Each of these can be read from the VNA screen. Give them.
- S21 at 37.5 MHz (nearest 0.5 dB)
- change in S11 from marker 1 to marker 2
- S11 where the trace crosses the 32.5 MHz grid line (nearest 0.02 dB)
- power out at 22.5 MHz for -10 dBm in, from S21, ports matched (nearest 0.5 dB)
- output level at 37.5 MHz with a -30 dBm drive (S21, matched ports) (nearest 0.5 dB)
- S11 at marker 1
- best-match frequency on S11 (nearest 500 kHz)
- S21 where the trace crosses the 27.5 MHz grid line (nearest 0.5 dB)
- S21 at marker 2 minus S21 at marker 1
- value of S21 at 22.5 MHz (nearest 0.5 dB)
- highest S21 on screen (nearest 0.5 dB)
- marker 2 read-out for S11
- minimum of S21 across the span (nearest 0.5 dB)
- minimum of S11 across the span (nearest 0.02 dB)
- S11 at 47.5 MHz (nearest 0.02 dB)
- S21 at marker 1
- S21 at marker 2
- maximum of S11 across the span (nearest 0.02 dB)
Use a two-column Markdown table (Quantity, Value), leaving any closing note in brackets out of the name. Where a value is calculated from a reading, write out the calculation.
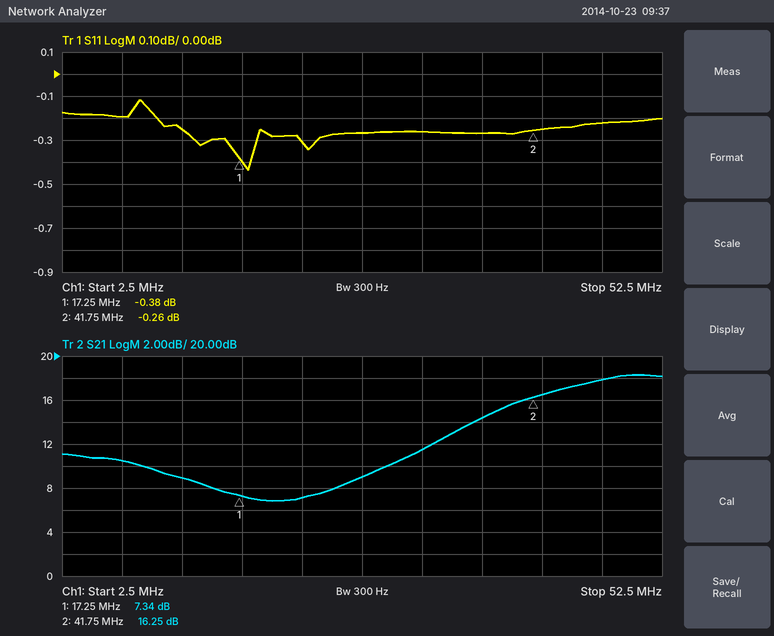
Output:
| Quantity | Value |
|---|---|
| S21 at 37.5 MHz | 14.5 dB |
| change in S11 from marker 1 to marker 2 | -0.26 − (-0.38) = 0.12 dB |
| S11 where the trace crosses the 32.5 MHz grid line | -0.26 dB |
| power out at 22.5 MHz for -10 dBm in, from S21, ports matched | -10 dBm + (7.0 dB) = -3.0 dBm |
| output level at 37.5 MHz with a -30 dBm drive (S21, matched ports) | -30 dBm + (14.5 dB) = -15.5 dBm |
| S11 at marker 1 | -0.38 dB |
| best-match frequency on S11 | 18.0 MHz |
| S21 where the trace crosses the 27.5 MHz grid line | 9.0 dB |
| S21 at marker 2 minus S21 at marker 1 | 16.25 − (7.34) = 8.91 dB |
| value of S21 at 22.5 MHz | 7.0 dB |
| highest S21 on screen | 18.5 dB |
| marker 2 read-out for S11 | -0.26 dB |
| minimum of S21 across the span | 7.0 dB |
| minimum of S11 across the span | -0.44 dB |
| S11 at 47.5 MHz | -0.22 dB |
| S21 at marker 1 | 7.34 dB |
| S21 at marker 2 | 16.25 dB |
| maximum of S11 across the span | -0.12 dB |
